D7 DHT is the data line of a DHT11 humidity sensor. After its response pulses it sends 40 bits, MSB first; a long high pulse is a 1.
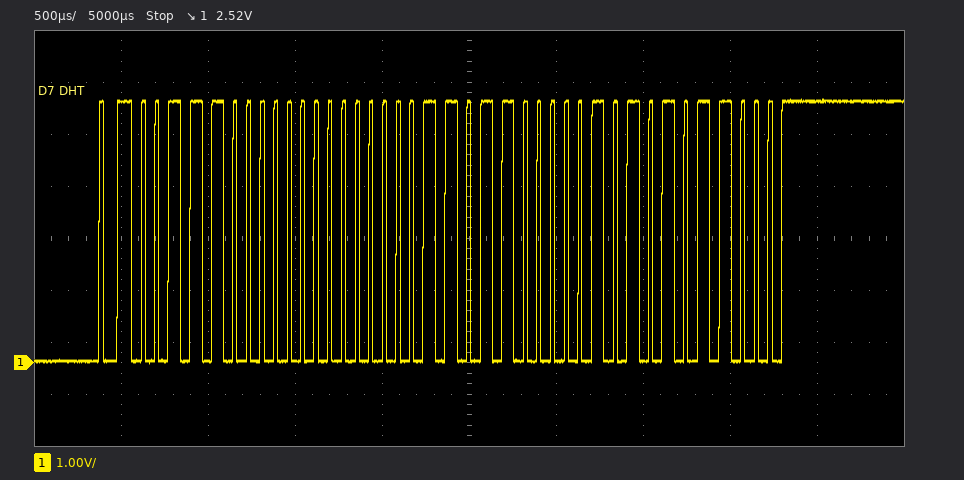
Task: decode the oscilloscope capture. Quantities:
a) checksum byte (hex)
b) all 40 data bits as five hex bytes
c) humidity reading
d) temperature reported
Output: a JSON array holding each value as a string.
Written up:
["0x58", "38 00 1B 05 58", "56 %", "27.5 °C"]
